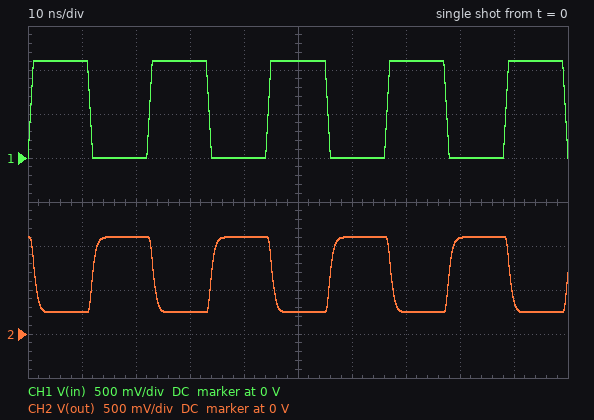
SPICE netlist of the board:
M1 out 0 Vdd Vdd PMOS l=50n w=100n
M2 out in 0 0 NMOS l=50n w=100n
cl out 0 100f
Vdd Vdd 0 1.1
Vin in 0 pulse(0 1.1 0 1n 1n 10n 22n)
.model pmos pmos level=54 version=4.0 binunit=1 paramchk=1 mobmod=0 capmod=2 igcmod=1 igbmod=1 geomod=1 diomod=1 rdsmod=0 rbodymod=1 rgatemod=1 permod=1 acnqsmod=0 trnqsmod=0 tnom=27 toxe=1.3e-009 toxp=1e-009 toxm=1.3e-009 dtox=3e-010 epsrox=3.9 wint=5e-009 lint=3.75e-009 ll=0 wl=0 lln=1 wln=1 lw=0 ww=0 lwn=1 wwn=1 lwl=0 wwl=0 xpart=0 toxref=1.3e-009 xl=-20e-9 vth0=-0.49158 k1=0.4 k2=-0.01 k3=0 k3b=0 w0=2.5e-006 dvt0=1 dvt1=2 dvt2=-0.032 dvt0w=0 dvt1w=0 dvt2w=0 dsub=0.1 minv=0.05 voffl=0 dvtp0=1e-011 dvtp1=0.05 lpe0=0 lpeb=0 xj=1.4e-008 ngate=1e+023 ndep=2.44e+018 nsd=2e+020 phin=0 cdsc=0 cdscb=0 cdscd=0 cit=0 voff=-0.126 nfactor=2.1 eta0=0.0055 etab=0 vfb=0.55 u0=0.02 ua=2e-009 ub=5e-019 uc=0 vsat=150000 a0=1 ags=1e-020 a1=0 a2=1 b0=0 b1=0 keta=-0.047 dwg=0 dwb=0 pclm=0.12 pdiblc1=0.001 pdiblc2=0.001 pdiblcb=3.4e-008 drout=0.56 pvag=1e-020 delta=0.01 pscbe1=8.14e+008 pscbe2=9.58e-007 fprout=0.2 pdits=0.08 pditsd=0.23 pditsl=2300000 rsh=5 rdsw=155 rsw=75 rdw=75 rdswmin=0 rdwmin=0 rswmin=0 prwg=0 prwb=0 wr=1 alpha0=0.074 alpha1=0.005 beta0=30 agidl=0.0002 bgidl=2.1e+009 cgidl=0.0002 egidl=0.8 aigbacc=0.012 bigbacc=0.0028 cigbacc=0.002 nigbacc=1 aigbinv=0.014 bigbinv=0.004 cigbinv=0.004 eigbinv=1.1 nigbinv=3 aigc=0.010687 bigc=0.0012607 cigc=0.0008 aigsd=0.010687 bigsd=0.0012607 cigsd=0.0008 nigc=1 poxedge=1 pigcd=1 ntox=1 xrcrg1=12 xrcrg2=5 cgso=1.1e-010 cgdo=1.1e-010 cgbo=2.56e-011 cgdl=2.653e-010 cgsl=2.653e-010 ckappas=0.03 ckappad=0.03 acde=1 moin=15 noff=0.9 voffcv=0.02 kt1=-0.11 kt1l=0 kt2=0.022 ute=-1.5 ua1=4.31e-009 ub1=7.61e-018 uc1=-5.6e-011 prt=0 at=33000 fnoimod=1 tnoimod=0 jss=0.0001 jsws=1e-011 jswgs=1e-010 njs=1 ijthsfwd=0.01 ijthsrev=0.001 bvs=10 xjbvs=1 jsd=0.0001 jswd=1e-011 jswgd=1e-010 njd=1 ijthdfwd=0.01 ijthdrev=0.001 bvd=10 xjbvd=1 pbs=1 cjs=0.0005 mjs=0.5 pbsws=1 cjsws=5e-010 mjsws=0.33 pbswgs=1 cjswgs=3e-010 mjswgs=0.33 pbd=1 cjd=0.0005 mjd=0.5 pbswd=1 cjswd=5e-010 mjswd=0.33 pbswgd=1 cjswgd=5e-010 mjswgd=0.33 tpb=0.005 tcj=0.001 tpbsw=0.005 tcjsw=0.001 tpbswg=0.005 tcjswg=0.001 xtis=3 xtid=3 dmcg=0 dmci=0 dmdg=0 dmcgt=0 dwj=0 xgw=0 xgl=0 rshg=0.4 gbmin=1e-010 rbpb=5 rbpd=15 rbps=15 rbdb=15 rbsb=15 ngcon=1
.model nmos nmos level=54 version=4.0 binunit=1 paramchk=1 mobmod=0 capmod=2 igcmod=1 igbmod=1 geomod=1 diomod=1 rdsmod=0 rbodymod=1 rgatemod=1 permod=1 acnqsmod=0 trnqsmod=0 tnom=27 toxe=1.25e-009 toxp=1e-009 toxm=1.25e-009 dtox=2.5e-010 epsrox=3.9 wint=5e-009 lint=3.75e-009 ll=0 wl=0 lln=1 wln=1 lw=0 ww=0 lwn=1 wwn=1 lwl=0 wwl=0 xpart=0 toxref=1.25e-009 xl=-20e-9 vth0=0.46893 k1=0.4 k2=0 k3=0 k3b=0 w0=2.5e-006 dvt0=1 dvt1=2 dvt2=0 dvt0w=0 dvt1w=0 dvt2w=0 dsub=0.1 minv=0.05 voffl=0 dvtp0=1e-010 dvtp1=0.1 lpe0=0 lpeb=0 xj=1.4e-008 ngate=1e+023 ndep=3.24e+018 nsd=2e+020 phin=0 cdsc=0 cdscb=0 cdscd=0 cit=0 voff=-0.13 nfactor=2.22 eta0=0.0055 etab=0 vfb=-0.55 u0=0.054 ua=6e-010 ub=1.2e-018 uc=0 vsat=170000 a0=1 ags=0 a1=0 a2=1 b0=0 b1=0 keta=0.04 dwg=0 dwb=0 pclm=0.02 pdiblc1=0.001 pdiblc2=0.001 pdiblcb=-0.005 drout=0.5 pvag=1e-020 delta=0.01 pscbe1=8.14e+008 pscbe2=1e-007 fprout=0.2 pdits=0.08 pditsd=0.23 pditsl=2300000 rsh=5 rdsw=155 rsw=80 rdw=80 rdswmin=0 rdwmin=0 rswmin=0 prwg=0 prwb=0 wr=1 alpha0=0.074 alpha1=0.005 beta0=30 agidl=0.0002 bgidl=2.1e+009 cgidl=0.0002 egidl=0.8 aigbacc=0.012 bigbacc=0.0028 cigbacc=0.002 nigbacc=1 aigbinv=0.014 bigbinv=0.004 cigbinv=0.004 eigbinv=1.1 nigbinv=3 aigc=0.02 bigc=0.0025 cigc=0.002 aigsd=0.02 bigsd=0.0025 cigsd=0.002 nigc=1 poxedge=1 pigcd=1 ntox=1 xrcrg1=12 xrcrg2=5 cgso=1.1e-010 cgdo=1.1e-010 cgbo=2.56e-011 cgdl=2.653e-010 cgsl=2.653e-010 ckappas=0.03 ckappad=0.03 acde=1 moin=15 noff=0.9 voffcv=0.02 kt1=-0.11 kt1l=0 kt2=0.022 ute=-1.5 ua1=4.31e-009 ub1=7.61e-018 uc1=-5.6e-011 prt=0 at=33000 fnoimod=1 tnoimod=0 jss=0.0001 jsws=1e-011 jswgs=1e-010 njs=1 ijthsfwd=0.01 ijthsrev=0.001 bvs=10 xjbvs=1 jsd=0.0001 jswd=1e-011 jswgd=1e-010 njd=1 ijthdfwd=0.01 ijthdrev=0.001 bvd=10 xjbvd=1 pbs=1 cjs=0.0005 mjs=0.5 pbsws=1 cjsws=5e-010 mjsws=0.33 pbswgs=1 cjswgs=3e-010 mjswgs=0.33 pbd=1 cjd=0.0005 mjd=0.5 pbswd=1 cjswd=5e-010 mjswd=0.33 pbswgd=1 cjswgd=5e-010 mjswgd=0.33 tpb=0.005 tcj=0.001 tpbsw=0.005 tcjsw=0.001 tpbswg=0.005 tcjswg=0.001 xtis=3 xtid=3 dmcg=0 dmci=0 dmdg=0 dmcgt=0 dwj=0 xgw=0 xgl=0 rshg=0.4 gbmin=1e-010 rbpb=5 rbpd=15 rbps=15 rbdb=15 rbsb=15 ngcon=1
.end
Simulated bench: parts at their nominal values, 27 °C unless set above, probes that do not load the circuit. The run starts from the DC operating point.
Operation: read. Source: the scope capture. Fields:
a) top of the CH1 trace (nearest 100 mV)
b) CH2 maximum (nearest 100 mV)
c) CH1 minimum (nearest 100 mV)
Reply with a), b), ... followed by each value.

a) 1.1 V
b) 1.1 V
c) 0 V
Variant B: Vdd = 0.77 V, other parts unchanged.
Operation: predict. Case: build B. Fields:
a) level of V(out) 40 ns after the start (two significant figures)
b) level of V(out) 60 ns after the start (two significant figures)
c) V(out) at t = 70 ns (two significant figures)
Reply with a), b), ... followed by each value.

a) 770 mV
b) 760 mV
c) 80 mV
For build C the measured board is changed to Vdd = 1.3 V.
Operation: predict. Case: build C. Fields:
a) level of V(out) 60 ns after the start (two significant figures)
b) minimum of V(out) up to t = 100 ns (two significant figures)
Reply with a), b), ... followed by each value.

a) 1.3 V
b) 420 mV
